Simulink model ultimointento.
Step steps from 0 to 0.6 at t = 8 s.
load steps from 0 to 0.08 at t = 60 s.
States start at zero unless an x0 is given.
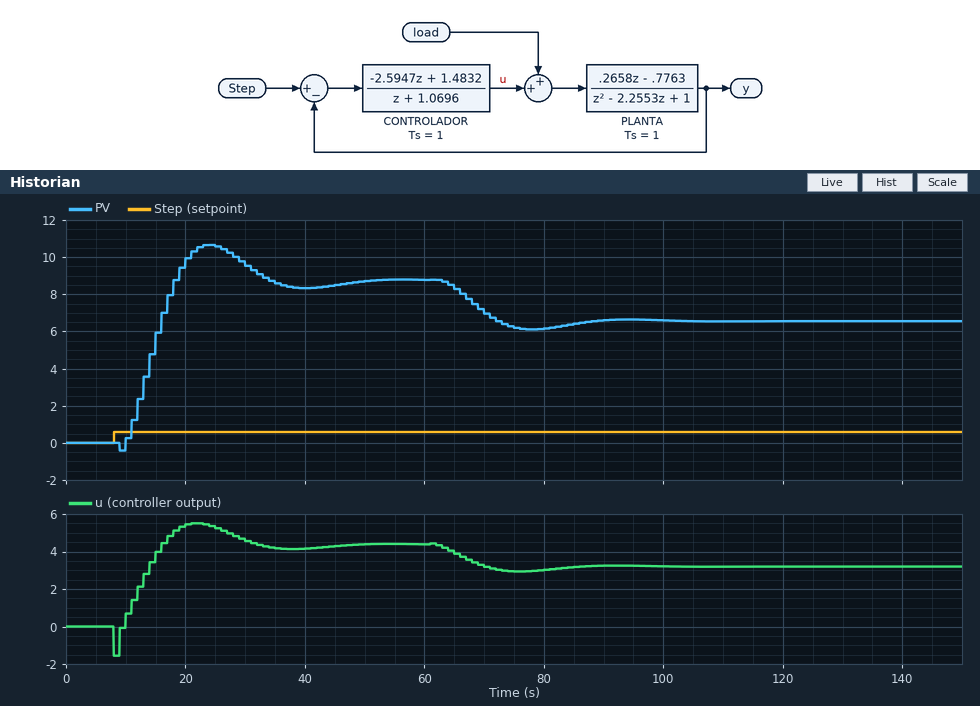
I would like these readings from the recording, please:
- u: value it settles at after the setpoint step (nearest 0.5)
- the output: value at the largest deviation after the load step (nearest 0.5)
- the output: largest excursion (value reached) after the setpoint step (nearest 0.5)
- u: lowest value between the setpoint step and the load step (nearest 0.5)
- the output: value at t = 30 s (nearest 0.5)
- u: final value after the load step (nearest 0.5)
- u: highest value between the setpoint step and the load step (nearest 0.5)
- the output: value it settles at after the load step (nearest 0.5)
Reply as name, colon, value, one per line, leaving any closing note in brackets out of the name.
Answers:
u: value it settles at after the setpoint step: 4.5
the output: value at the largest deviation after the load step: 6.0
the output: largest excursion (value reached) after the setpoint step: 10.5
u: lowest value between the setpoint step and the load step: -1.5
the output: value at t = 30 s: 9.5
u: final value after the load step: 3.0
u: highest value between the setpoint step and the load step: 5.5
the output: value it settles at after the load step: 6.5
